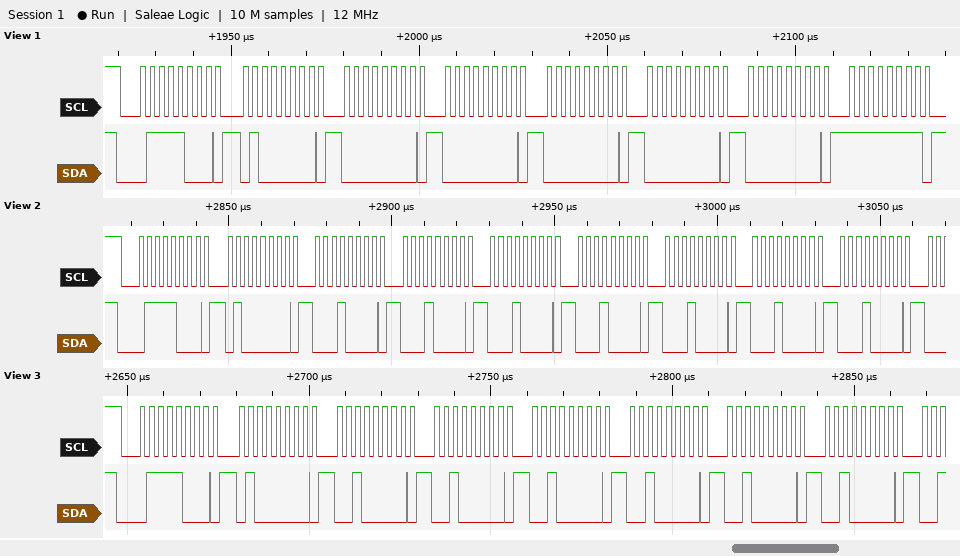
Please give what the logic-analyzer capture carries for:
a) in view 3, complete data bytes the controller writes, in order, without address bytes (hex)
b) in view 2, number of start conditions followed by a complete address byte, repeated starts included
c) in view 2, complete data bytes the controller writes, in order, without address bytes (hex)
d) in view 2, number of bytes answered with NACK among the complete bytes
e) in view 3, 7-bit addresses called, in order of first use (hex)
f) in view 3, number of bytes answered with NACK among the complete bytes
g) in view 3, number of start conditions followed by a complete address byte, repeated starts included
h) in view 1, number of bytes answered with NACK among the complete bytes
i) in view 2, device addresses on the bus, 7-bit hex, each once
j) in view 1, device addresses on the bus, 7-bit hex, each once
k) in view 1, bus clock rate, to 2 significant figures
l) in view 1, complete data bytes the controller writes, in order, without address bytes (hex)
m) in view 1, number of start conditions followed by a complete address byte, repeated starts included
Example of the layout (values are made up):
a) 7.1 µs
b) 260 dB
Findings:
a) 40 20 20 20 20 20 20
b) 1
c) 40 10 10 10 10 10 10 10
d) 0
e) 0x3C
f) 0
g) 1
h) 0
i) 0x3C
j) 0x3C
k) 400 kHz
l) 40 00 00 00 00 00 FF
m) 1
